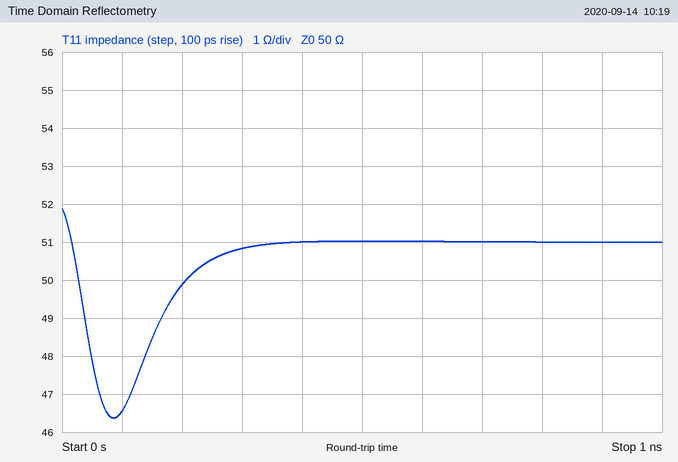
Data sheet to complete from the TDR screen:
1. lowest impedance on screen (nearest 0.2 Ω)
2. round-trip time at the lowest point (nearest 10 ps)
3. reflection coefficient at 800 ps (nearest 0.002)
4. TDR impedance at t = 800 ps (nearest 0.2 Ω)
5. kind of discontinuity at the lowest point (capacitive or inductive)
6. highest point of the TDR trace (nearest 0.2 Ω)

46.4 Ω
90 ps
+0.010
51.0 Ω
capacitive
51.8 Ω
